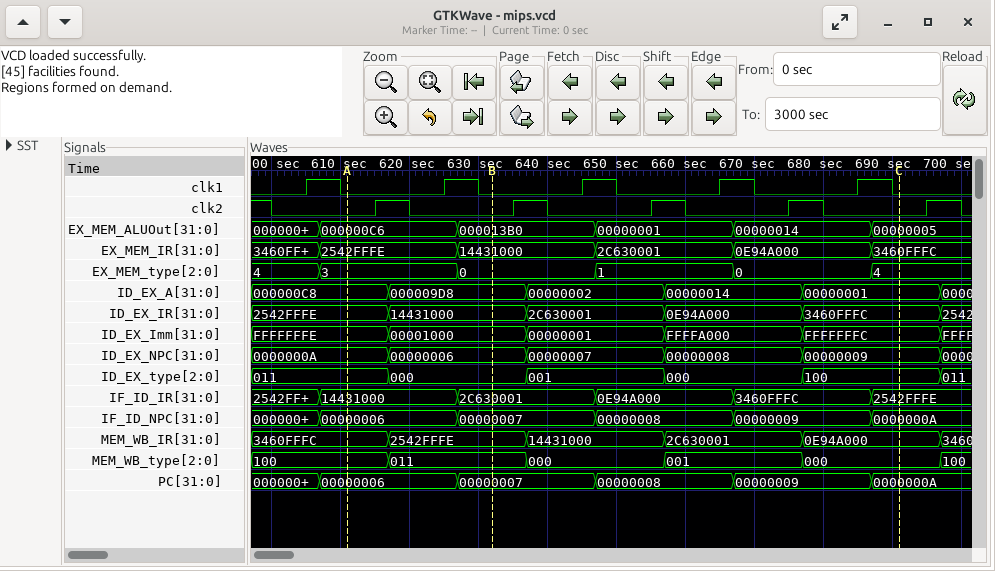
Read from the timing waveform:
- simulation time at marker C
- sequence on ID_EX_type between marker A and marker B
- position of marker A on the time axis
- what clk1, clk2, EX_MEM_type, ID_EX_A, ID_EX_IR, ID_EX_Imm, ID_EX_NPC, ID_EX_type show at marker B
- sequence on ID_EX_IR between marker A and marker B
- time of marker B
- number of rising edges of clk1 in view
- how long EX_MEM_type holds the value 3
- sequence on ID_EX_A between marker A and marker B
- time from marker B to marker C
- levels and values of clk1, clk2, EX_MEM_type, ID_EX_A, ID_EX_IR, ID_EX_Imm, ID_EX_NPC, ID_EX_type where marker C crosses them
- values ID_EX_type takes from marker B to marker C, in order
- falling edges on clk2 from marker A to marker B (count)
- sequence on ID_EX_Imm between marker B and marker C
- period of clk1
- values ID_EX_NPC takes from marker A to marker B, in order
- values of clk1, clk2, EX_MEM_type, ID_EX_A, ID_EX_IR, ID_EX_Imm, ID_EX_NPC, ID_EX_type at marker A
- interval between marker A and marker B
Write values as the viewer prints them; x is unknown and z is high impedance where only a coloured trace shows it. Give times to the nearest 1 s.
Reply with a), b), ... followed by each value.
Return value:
a) 691 s
b) 011, 000
c) 611 s
d) clk1=0, clk2=0, EX_MEM_type=0, ID_EX_A=000009D8, ID_EX_IR=14431000, ID_EX_Imm=00001000, ID_EX_NPC=00000006, ID_EX_type=000
e) 2542FFFE, 14431000
f) 632 s
g) 5
h) 20 s
i) 000000C8, 000009D8
j) 59 s
k) clk1=0, clk2=0, EX_MEM_type=4, ID_EX_A=00000001, ID_EX_IR=3460FFFC, ID_EX_Imm=FFFFFFFC, ID_EX_NPC=00000009, ID_EX_type=100
l) 000, 001, 000, 100
m) 1
n) 00001000, 00000001, FFFFA000, FFFFFFFC
o) 20 s
p) 0000000A, 00000006
q) clk1=0, clk2=0, EX_MEM_type=3, ID_EX_A=000000C8, ID_EX_IR=2542FFFE, ID_EX_Imm=FFFFFFFE, ID_EX_NPC=0000000A, ID_EX_type=011
r) 21 s
